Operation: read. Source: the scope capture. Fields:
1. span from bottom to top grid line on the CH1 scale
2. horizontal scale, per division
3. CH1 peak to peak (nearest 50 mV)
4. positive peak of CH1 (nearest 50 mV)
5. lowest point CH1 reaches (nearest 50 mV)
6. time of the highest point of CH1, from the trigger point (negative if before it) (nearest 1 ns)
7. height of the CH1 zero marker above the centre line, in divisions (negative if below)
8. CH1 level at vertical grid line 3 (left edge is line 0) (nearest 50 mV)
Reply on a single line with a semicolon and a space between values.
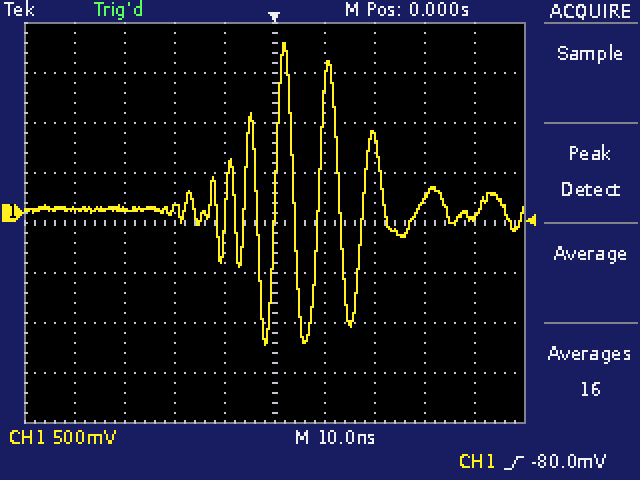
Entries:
4 V; 10 ns; 3.00 V; 1.70 V; -1.30 V; +2 ns; +0.2 div; 50 mV
